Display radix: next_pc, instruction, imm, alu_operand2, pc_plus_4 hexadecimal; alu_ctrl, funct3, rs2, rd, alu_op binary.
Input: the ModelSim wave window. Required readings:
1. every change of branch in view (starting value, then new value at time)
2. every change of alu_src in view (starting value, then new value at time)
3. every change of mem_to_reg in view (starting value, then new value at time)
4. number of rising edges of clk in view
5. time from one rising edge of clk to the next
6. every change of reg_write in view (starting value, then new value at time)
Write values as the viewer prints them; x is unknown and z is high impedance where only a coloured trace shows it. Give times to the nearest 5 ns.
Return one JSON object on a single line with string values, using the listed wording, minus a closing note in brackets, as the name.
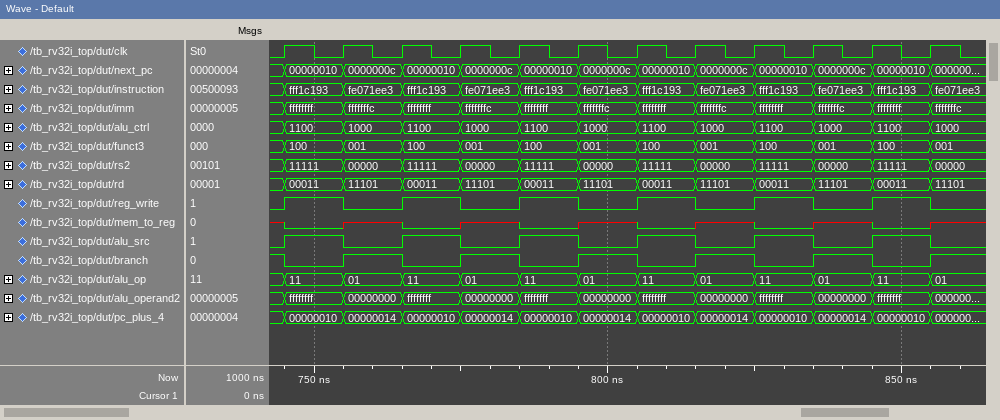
{"every change of branch in view": "1, 0 at 745 ns, 1 at 755 ns, 0 at 765 ns, 1 at 775 ns, 0 at 785 ns, 1 at 795 ns, 0 at 805 ns, 1 at 815 ns, 0 at 825 ns, 1 at 835 ns, 0 at 845 ns, 1 at 855 ns", "every change of alu_src in view": "0, 1 at 745 ns, 0 at 755 ns, 1 at 765 ns, 0 at 775 ns, 1 at 785 ns, 0 at 795 ns, 1 at 805 ns, 0 at 815 ns, 1 at 825 ns, 0 at 835 ns, 1 at 845 ns, 0 at 855 ns", "every change of mem_to_reg in view": "x, 0 at 745 ns, x at 755 ns, 0 at 765 ns, x at 775 ns, 0 at 785 ns, x at 795 ns, 0 at 805 ns, x at 815 ns, 0 at 825 ns, x at 835 ns, 0 at 845 ns, x at 855 ns", "number of rising edges of clk in view": "12", "time from one rising edge of clk to the next": "10 ns", "every change of reg_write in view": "0, 1 at 745 ns, 0 at 755 ns, 1 at 765 ns, 0 at 775 ns, 1 at 785 ns, 0 at 795 ns, 1 at 805 ns, 0 at 815 ns, 1 at 825 ns, 0 at 835 ns, 1 at 845 ns, 0 at 855 ns"}
